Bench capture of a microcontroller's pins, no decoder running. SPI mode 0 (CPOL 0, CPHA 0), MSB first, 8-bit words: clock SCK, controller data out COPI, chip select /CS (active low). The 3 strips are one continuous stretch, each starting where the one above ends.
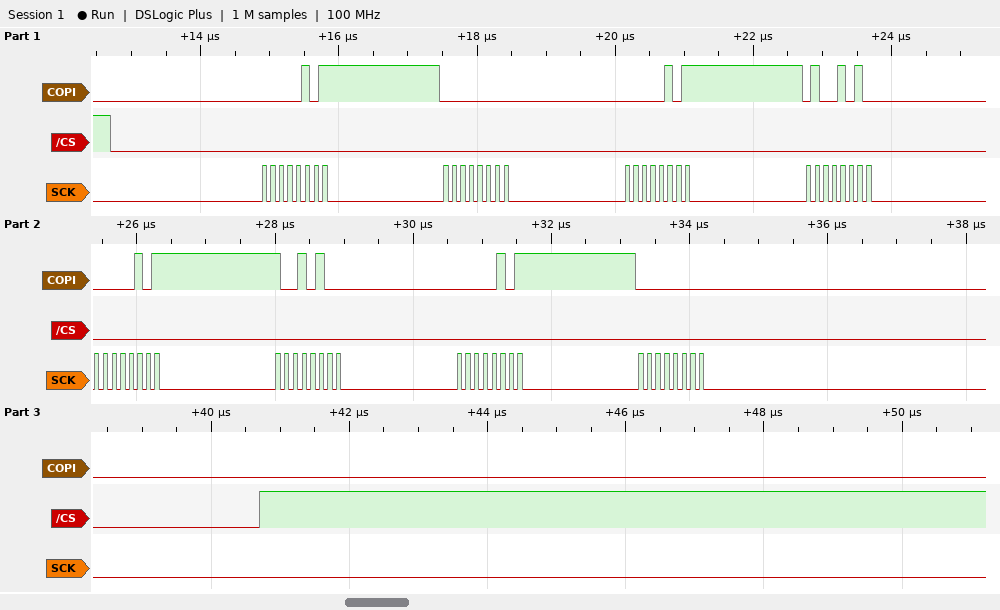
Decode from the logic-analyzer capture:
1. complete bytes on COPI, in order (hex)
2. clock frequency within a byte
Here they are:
05 00 05 4A 05 94 05 00
8 MHz
